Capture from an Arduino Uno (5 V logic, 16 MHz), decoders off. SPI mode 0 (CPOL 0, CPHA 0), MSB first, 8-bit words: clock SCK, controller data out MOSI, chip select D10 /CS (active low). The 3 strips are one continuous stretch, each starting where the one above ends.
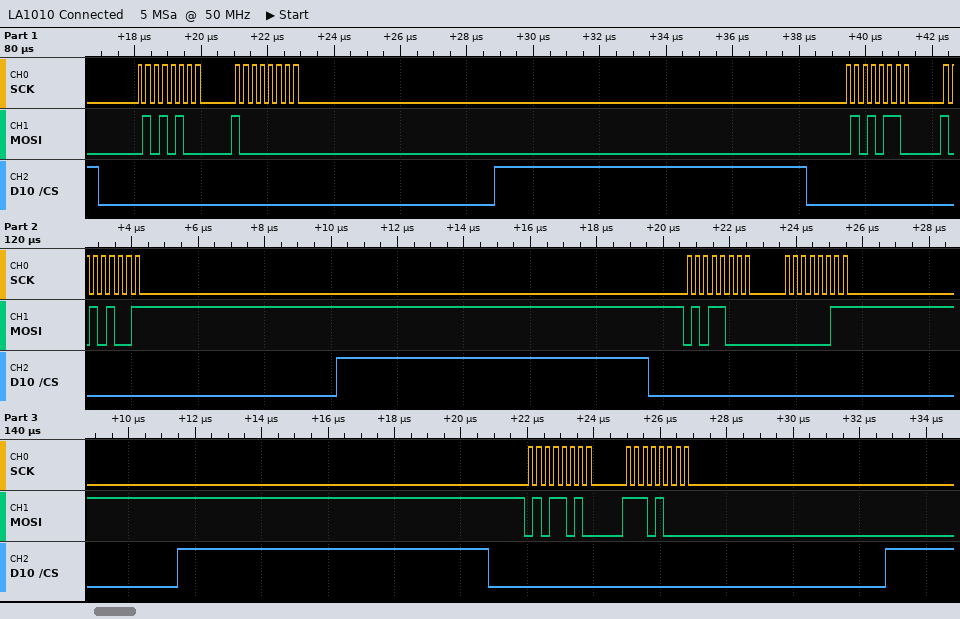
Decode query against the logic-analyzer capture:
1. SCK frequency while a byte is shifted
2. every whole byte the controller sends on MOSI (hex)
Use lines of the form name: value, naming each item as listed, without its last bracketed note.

SCK frequency while a byte is shifted: 4 MHz
every whole byte the controller sends on MOSI: 54 80 56 A9 58 03 5A E8
